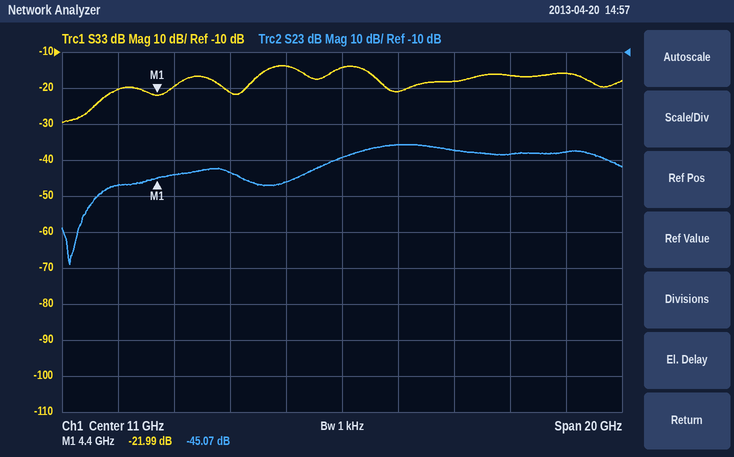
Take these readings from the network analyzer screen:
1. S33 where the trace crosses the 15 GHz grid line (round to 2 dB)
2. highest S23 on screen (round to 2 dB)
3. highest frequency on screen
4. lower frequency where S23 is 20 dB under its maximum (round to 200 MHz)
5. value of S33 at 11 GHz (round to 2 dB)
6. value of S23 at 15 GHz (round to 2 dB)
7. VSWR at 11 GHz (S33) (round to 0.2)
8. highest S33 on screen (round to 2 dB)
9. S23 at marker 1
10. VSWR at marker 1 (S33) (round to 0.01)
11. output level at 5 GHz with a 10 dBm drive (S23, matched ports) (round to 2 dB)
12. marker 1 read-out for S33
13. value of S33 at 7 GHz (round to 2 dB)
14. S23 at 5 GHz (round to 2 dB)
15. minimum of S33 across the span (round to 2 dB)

-18 dB
-36 dB
21 GHz
1.8 GHz
-14 dB
-38 dB
1.4
-14 dB
-45.07 dB
1.17
-34 dBm
-21.99 dB
-22 dB
-44 dB
-30 dB
